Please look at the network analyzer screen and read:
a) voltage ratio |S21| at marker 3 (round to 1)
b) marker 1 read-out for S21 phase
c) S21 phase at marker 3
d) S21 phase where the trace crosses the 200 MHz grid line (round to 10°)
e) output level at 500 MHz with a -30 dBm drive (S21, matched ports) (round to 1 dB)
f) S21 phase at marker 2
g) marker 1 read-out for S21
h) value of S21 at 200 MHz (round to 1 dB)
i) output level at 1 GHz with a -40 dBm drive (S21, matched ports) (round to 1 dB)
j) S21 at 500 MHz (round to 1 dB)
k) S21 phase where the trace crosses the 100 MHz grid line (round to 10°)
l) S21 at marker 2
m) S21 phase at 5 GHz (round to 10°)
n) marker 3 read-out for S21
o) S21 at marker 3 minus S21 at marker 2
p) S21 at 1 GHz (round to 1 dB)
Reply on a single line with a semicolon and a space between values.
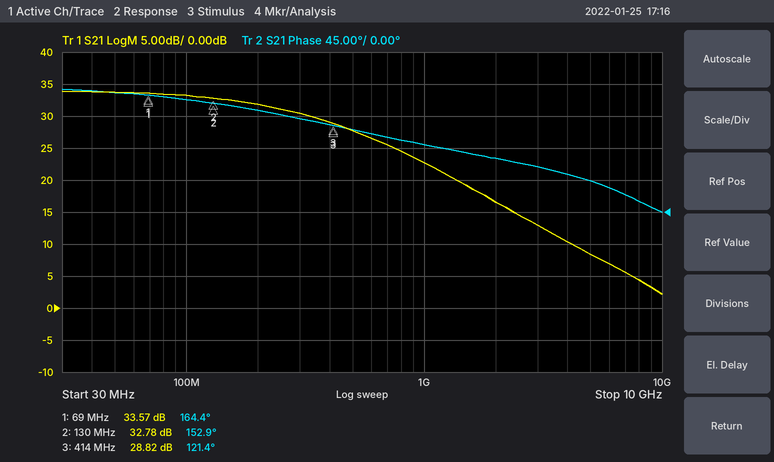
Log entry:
28; 164.4°; 121.4°; 140°; -2 dBm; 152.9°; 33.57 dB; 32 dB; -17 dBm; 28 dB; 160°; 32.78 dB; 40°; 28.82 dB; -3.96 dB; 23 dB
